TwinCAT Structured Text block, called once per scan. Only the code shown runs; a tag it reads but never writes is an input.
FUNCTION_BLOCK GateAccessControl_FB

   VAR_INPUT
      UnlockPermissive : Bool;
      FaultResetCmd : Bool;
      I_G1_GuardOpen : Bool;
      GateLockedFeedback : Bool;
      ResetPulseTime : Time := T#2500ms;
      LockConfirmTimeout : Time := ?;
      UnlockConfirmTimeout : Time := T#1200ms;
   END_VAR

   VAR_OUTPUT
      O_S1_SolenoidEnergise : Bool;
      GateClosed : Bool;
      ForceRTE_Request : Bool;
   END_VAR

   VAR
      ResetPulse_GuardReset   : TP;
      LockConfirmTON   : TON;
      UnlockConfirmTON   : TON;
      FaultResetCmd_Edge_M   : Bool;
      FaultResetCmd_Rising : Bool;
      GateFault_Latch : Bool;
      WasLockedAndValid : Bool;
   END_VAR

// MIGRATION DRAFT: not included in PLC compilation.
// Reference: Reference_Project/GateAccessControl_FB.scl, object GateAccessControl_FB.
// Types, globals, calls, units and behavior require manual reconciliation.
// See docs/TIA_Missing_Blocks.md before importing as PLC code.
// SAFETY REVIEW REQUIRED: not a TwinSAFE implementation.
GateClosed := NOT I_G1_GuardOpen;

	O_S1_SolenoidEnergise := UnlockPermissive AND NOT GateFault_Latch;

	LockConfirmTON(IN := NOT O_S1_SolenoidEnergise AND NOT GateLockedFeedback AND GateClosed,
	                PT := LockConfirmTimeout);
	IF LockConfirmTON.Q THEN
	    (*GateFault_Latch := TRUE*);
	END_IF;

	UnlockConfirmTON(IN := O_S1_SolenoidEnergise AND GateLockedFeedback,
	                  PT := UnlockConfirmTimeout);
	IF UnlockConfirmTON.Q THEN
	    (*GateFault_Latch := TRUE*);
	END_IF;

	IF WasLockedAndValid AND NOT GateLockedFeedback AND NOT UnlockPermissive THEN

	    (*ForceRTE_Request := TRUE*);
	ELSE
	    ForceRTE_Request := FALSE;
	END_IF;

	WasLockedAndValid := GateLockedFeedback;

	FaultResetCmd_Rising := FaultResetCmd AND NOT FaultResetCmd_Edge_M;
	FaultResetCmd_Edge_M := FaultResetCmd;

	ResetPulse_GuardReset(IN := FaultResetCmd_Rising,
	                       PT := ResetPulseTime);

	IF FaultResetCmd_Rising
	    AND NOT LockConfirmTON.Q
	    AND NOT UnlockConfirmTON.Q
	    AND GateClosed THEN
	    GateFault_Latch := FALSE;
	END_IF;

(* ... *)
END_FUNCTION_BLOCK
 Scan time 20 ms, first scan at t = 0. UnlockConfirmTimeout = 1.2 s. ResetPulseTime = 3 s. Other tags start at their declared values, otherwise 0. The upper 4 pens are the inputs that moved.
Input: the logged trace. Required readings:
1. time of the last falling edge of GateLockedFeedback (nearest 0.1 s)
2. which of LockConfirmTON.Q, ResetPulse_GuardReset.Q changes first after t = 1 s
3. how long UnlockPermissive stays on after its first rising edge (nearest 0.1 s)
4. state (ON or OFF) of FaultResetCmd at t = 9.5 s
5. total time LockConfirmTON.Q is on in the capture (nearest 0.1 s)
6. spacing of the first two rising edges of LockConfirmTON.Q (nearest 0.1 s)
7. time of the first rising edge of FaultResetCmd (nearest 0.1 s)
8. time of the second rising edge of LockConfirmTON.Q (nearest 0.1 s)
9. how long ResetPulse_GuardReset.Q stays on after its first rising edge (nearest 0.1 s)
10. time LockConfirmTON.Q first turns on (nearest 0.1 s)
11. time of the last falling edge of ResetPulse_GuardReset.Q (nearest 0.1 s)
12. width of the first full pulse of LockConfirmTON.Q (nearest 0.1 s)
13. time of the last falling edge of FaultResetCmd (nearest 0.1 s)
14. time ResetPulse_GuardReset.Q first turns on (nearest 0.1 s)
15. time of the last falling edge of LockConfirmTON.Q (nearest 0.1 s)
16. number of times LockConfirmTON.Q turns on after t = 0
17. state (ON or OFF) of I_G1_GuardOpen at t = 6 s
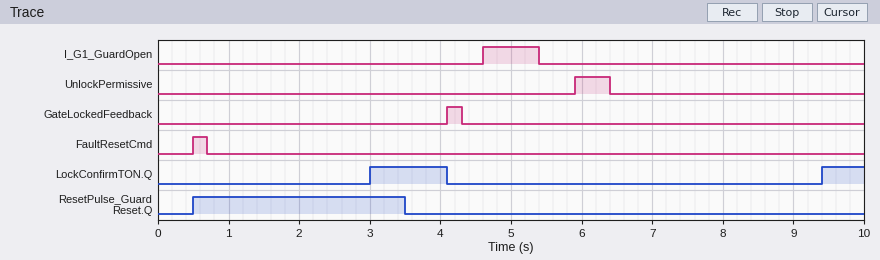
4.3 s
LockConfirmTON.Q
0.5 s
OFF
1.7 s
6.4 s
0.5 s
9.4 s
3.0 s
3.0 s
3.5 s
1.1 s
0.7 s
0.5 s
4.1 s
2
OFF
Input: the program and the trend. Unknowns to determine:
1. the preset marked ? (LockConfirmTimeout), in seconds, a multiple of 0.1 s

3.0 s
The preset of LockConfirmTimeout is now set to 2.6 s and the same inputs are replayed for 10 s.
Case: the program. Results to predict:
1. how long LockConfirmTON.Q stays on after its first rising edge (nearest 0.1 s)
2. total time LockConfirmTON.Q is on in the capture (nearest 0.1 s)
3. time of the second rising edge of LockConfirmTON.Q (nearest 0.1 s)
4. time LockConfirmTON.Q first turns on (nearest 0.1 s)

1.5 s
2.5 s
9.0 s
2.6 s
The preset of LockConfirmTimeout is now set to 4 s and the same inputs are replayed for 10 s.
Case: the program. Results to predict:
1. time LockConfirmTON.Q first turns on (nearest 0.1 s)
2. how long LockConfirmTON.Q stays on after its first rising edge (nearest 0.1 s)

4.0 s
0.1 s
